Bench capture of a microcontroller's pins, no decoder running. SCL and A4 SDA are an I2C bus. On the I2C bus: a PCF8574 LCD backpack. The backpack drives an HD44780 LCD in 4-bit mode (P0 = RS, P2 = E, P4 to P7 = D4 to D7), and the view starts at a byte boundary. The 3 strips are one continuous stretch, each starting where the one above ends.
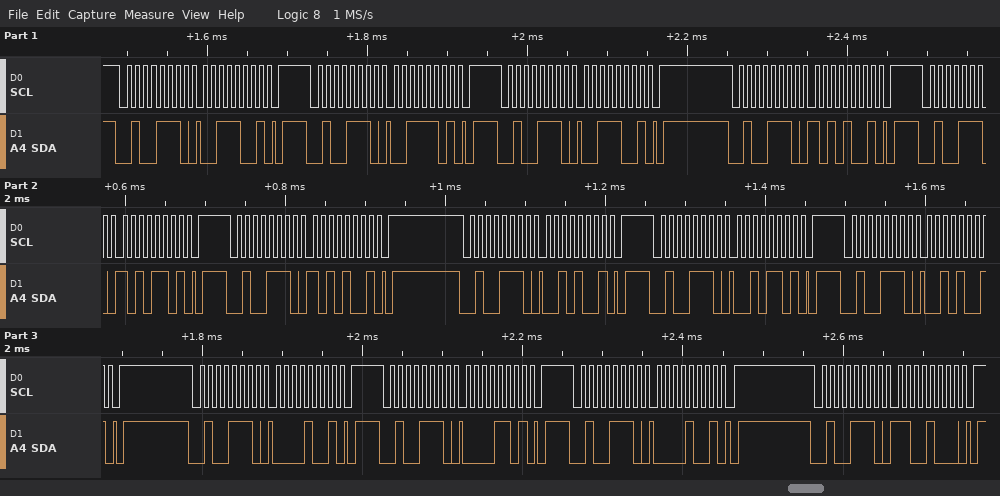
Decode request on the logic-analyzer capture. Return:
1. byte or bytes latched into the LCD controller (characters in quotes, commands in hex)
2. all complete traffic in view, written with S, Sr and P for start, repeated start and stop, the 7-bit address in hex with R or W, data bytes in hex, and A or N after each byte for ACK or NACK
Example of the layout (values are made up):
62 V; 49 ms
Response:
':' ' '; S 27W A 39 A P S 27W A 3D A P S 27W A 39 A P S 27W A A9 A P S 27W A AD A P S 27W A A9 A P S 27W A 29 A P S 27W A 2D A P S 27W A 29 A P S 27W A 09 A P S 27W A 0D A P S 27W A 09 A P S 27W A C8 A P
